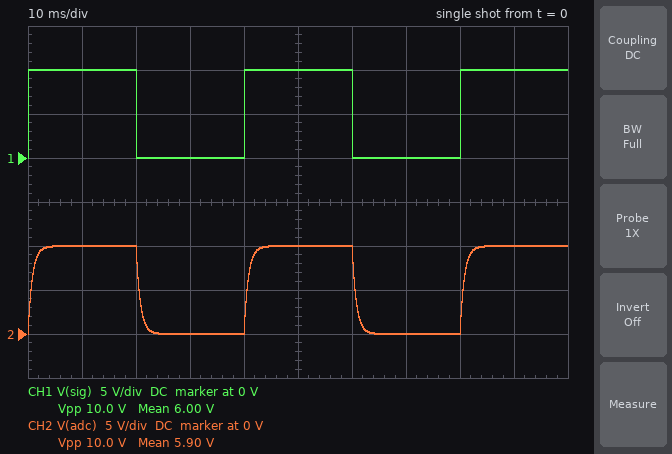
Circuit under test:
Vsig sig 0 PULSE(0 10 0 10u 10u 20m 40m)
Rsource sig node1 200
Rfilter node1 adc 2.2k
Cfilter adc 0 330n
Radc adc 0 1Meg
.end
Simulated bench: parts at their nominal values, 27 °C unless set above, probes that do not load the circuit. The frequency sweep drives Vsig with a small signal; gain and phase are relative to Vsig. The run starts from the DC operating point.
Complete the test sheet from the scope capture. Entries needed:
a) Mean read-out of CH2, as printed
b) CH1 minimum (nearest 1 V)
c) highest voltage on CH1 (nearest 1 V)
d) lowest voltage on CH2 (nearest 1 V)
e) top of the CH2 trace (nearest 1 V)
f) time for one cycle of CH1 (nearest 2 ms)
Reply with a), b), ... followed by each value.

a) 5.90 V
b) 0 V
c) 10 V
d) 0 V
e) 10 V
f) 40 ms
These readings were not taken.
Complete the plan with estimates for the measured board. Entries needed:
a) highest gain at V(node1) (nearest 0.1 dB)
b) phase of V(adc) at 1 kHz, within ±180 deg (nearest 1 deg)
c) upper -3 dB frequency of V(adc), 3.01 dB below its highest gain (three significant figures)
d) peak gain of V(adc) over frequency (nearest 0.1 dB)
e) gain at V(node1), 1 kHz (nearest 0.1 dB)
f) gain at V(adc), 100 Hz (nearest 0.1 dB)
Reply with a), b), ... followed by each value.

a) 0 dB
b) -79 deg
c) 201 Hz
d) 0 dB
e) -0.7 dB
f) -1.0 dB
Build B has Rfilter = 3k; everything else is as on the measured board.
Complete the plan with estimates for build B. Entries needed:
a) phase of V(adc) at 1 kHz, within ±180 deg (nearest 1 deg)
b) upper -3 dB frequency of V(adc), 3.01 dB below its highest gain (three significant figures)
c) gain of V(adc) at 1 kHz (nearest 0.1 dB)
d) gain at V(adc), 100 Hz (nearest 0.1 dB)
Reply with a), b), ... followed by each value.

a) -81 deg
b) 151 Hz
c) -16.5 dB
d) -1.6 dB
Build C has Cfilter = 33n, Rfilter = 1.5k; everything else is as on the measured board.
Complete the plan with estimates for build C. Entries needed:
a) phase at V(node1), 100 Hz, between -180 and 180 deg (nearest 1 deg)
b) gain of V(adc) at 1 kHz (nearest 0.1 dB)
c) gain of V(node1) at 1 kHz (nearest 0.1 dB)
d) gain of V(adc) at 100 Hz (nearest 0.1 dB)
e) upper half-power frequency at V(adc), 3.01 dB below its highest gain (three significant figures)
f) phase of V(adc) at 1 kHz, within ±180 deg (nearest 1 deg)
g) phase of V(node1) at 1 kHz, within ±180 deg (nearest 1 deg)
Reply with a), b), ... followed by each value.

a) 0 deg
b) -0.5 dB
c) -0.1 dB
d) 0 dB
e) 2.84 kHz
f) -19 deg
g) -2 deg
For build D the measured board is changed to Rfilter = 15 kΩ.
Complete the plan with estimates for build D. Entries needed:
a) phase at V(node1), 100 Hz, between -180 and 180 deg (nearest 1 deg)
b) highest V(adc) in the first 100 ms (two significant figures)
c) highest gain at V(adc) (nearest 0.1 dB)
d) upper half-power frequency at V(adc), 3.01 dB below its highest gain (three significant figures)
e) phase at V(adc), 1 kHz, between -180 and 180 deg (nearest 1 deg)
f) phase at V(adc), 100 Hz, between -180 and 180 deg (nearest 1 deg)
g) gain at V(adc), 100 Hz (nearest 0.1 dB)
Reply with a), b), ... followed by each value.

a) 0 deg
b) 9.7 V
c) -0.1 dB
d) 32.2 Hz
e) -88 deg
f) -72 deg
g) -10.4 dB
